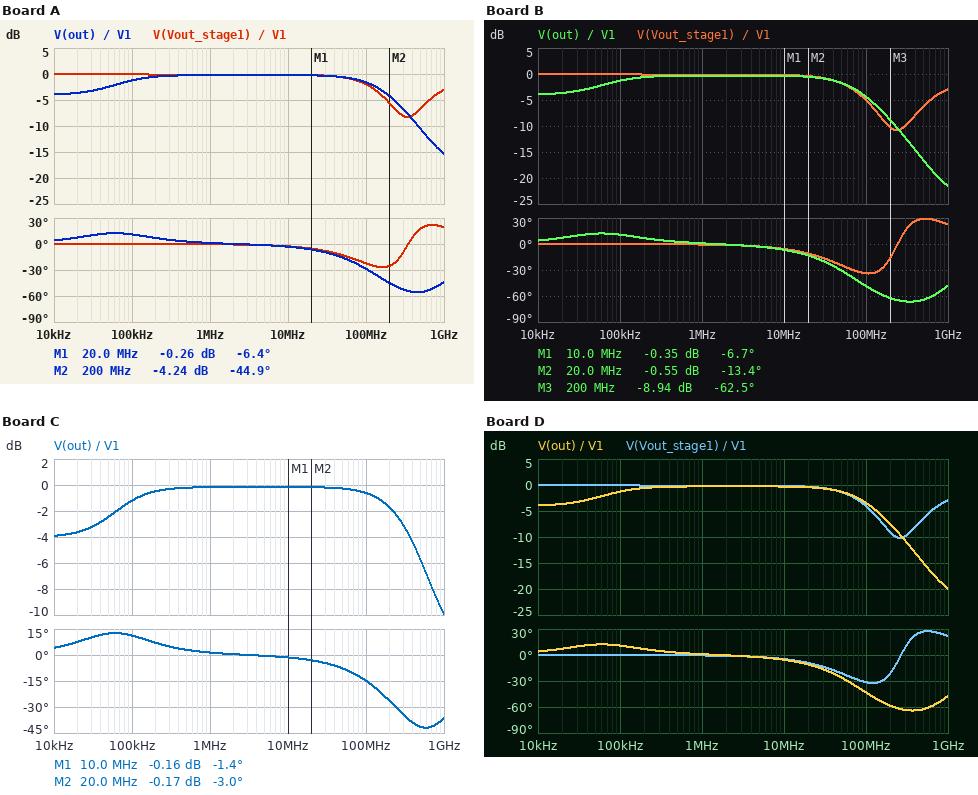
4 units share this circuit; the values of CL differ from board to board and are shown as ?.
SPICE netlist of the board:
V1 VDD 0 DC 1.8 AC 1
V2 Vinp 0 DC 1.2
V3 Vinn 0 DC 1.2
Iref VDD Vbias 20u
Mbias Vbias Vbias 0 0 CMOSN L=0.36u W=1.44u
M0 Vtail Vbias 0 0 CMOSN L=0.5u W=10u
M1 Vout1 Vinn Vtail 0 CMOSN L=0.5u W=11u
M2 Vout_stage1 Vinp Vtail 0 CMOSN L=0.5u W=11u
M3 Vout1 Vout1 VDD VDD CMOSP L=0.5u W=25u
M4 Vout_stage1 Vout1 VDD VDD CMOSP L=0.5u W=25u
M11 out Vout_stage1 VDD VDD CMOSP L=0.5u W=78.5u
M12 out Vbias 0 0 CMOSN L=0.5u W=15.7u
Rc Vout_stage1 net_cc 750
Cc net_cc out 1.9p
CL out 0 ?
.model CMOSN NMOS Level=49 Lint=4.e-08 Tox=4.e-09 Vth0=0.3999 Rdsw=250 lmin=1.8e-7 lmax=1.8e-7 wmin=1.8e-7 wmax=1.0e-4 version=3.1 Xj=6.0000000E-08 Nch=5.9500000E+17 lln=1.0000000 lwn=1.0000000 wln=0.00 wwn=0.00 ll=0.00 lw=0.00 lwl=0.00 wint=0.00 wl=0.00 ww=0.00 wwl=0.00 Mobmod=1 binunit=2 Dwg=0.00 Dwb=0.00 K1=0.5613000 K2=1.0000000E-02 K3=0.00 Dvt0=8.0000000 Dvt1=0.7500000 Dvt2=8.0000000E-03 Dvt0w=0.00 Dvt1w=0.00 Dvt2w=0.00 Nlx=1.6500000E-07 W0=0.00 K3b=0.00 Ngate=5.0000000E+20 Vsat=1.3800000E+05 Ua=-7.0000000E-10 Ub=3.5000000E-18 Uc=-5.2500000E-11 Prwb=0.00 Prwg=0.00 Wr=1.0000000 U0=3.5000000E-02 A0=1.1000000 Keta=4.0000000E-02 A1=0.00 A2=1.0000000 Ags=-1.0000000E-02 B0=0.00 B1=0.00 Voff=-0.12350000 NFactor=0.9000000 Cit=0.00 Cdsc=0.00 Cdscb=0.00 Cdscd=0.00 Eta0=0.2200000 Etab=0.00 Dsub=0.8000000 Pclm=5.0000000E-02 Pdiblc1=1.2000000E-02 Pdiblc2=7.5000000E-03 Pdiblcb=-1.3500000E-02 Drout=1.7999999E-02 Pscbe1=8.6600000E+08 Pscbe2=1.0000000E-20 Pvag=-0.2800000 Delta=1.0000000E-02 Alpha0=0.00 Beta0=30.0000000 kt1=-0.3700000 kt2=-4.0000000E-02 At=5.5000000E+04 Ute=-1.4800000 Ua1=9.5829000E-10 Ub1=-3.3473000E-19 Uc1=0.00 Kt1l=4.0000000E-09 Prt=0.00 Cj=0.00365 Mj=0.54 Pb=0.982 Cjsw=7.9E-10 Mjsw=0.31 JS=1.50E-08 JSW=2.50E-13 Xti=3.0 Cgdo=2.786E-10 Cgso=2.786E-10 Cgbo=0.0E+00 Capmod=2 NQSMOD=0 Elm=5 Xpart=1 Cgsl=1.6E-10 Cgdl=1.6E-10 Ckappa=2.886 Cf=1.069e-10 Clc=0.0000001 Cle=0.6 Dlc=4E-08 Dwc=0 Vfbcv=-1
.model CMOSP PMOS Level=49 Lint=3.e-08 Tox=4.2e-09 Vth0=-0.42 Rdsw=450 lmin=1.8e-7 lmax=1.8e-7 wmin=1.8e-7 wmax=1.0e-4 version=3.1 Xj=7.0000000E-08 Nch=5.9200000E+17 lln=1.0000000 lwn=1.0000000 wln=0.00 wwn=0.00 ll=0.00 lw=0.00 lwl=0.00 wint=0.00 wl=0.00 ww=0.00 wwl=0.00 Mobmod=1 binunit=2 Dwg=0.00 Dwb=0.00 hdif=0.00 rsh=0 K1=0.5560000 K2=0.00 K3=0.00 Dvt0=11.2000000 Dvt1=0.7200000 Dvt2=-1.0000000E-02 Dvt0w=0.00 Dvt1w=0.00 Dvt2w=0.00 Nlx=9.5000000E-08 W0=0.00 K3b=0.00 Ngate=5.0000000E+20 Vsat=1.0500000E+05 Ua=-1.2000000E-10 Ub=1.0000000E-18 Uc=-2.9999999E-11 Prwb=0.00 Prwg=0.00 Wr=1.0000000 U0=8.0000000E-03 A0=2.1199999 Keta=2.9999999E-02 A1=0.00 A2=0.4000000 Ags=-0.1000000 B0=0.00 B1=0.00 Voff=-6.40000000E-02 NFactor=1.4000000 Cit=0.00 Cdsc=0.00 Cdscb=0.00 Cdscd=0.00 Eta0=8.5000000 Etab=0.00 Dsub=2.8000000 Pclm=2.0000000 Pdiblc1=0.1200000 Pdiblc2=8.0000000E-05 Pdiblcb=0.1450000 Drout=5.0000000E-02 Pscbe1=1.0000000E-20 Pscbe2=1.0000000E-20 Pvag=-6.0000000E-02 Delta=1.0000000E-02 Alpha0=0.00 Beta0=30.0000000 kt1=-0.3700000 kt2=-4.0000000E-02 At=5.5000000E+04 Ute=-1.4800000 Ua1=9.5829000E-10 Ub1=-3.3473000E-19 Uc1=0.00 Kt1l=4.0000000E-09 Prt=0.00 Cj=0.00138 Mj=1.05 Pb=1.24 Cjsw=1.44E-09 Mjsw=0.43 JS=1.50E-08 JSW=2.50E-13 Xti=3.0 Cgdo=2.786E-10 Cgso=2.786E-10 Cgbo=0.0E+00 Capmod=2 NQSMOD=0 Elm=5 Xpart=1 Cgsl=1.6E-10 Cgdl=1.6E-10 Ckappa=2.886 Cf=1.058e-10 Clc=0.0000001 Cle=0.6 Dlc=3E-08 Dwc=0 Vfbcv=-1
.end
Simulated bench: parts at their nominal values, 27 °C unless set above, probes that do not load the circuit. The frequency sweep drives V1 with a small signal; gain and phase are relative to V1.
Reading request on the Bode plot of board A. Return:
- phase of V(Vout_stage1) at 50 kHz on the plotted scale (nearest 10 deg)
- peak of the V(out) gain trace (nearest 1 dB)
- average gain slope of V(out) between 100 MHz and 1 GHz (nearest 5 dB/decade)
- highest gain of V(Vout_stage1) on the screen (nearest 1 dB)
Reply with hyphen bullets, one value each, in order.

- 0 deg
- 0 dB
- -15 dB/decade
- 0 dB
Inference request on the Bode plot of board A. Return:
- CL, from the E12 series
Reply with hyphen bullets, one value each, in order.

- 1.5 pF
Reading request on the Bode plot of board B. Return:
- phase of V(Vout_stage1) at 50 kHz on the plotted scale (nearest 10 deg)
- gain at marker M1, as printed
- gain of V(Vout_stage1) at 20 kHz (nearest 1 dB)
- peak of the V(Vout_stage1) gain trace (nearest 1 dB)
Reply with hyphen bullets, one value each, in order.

- 0 deg
- -0.35 dB
- 0 dB
- 0 dB
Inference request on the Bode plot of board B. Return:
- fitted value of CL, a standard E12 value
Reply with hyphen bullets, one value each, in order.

- 3.3 pF
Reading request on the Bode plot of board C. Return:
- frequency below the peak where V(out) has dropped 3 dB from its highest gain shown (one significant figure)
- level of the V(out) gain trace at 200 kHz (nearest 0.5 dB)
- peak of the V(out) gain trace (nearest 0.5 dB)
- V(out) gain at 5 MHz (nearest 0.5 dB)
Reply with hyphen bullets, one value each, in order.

- 30 kHz
- -0.5 dB
- 0 dB
- 0 dB
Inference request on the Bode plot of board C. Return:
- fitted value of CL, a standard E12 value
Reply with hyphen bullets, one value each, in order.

- 680 fF
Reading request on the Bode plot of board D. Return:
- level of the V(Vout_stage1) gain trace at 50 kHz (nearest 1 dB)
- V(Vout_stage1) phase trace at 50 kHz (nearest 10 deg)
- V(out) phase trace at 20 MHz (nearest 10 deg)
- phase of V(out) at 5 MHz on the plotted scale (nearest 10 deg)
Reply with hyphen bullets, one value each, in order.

- 0 dB
- 0 deg
- -10 deg
- 0 deg
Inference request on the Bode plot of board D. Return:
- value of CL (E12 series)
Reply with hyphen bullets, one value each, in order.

- 2.7 pF
